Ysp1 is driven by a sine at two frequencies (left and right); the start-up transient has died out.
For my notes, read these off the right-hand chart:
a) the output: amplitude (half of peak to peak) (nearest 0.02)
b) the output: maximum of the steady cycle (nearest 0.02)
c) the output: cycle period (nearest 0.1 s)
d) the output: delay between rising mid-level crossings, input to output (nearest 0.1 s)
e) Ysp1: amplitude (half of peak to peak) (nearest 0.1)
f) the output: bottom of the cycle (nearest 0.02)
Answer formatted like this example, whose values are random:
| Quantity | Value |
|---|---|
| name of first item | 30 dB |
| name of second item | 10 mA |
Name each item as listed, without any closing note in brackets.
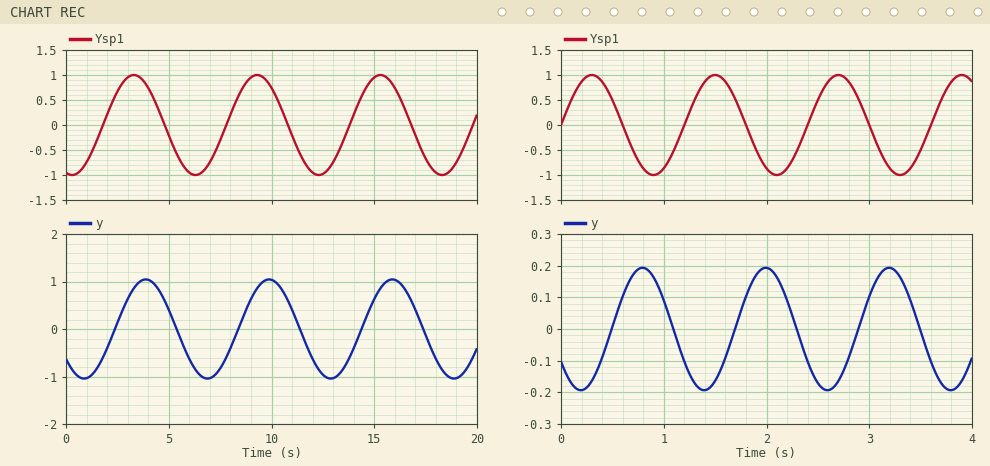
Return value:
| Quantity | Value |
|---|---|
| the output: amplitude (half of peak to peak) | 0.20 |
| the output: maximum of the steady cycle | 0.20 |
| the output: cycle period | 1.2 s |
| the output: delay between rising mid-level crossings, input to output | 0.5 s |
| Ysp1: amplitude (half of peak to peak) | 1.0 |
| the output: bottom of the cycle | -0.20 |
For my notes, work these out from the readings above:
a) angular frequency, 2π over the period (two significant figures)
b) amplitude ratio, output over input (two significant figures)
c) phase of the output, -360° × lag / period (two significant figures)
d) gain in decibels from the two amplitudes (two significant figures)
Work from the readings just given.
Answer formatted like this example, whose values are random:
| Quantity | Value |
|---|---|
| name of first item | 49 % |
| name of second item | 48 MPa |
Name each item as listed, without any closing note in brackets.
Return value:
| Quantity | Value |
|---|---|
| angular frequency, 2π over the period | 5.2 rad/s |
| amplitude ratio, output over input | 0.20 |
| phase of the output, -360° × lag / period | -150° |
| gain in decibels from the two amplitudes | -14 dB |
